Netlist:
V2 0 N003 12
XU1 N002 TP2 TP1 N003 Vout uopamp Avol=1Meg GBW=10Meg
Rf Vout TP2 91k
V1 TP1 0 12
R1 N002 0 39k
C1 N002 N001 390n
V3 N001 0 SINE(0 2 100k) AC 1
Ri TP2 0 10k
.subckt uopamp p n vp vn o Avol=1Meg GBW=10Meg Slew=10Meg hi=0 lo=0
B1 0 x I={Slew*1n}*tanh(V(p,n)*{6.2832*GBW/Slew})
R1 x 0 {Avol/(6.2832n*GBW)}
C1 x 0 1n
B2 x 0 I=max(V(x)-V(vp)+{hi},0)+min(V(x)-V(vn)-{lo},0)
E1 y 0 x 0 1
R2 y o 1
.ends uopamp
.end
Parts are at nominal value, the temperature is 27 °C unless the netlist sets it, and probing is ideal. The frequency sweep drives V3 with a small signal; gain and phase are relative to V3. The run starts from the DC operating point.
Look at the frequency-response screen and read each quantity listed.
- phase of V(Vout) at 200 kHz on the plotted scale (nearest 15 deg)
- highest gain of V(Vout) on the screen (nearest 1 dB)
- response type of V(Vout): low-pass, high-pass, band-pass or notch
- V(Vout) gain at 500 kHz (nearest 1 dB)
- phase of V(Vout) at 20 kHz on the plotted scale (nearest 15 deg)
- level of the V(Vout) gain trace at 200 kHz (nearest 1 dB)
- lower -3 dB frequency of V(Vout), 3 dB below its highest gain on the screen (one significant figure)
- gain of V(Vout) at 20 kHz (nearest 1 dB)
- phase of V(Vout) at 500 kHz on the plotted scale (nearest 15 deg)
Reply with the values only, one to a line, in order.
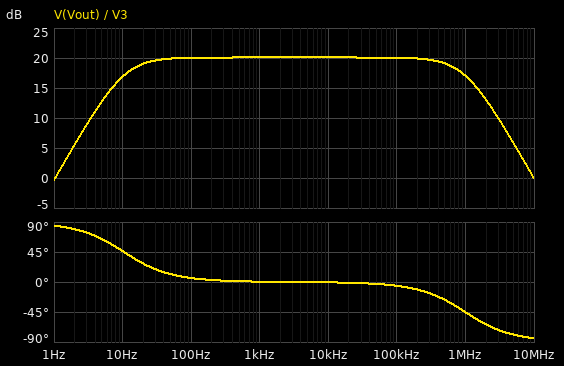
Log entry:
-15 deg
20 dB
band-pass
19 dB
0 deg
20 dB
10 Hz
20 dB
-30 deg
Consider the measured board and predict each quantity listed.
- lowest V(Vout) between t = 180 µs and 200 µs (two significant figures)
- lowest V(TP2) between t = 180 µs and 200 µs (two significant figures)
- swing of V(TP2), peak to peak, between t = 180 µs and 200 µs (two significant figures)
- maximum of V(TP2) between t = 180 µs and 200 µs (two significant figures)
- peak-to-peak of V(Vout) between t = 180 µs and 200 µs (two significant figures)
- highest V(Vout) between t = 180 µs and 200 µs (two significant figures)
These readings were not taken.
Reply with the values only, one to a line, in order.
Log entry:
-12 V
-1.2 V
2.4 V
1.2 V
24 V
12 V
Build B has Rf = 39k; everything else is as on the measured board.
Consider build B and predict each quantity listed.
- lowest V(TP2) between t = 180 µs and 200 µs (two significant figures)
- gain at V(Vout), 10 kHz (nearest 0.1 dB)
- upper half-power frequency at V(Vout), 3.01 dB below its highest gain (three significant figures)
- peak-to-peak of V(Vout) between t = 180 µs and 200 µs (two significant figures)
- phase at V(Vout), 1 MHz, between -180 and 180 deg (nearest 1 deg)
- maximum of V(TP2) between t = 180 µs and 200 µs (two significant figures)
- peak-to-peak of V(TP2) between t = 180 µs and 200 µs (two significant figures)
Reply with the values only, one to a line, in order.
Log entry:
-2.0 V
13.8 dB
2.04 MHz
20 V
-26 deg
2.0 V
4.0 V
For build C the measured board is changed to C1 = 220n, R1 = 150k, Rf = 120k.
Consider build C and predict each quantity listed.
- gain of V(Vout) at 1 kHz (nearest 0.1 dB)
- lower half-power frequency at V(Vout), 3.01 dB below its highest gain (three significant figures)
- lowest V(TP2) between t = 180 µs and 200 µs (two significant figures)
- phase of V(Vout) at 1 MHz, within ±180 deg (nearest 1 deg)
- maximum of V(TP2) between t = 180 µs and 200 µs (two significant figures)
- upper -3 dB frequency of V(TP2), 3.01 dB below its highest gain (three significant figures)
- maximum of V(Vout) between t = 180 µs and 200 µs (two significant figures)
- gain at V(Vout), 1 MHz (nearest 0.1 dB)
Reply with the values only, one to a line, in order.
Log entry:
22.3 dB
4.82 Hz
-920 mV
-52 deg
920 mV
769 kHz
12 V
18.0 dB
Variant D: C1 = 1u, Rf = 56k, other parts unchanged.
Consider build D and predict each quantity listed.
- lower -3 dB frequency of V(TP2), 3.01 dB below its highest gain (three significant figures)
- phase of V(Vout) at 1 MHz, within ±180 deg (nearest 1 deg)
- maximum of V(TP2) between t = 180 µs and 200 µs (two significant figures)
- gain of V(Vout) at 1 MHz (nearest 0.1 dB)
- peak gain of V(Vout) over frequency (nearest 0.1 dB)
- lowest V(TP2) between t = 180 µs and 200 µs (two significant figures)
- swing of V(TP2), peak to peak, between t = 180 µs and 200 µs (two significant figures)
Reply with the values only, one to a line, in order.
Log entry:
4.08 Hz
-33 deg
1.8 V
14.8 dB
16.4 dB
-1.8 V
3.6 V
